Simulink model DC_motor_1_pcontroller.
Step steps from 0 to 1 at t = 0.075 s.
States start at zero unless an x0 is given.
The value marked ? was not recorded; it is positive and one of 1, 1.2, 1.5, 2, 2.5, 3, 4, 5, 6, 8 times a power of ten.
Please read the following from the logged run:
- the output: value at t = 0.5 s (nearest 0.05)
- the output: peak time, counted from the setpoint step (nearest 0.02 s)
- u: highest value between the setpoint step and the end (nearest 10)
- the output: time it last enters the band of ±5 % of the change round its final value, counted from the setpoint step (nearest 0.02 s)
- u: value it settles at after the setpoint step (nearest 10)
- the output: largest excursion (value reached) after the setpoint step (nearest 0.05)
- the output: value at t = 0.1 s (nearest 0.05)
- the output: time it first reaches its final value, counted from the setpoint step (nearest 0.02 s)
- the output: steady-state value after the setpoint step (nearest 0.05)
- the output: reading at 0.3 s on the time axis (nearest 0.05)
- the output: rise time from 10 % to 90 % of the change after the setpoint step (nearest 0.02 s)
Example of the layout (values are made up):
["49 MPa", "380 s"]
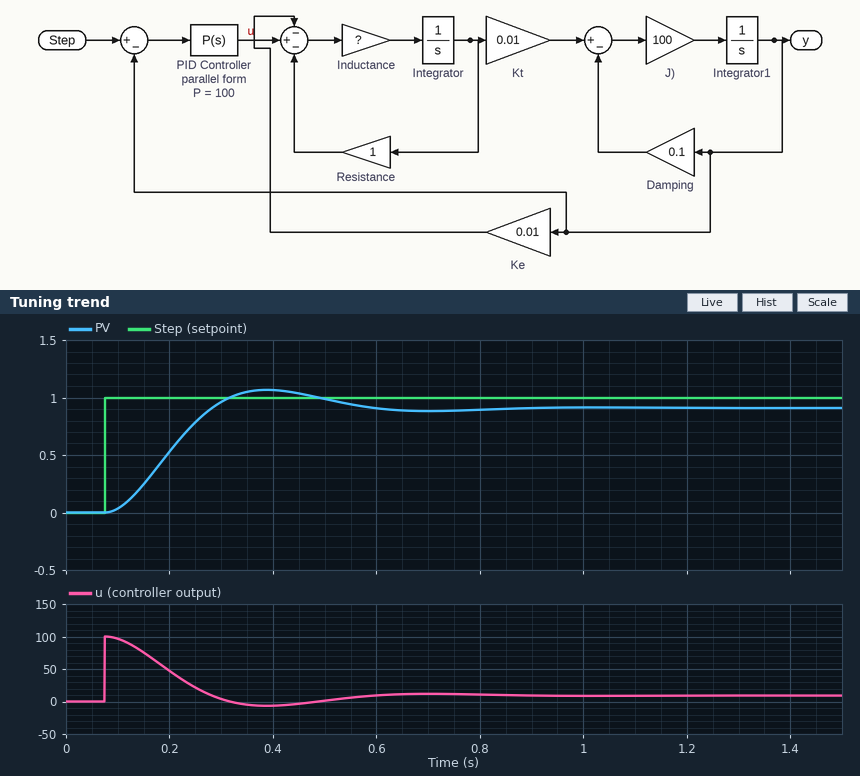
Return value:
["1.00", "0.32 s", "100", "0.46 s", "10", "1.05", "0.05", "0.20 s", "0.90", "0.95", "0.14 s"]
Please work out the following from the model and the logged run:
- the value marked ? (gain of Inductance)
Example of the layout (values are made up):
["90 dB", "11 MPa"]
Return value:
["1.2"]
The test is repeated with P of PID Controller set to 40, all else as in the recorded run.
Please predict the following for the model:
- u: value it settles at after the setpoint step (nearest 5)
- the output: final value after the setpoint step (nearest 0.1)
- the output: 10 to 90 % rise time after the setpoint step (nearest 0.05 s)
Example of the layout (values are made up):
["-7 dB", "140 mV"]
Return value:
["10", "0.8", "0.30 s"]
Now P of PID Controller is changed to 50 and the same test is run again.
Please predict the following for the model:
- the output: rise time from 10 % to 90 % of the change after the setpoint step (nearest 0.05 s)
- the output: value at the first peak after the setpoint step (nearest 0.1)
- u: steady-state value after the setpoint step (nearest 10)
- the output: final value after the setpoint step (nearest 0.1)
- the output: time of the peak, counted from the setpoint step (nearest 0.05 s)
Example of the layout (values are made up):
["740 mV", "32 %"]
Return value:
["0.25 s", "0.9", "10", "0.8", "0.50 s"]
